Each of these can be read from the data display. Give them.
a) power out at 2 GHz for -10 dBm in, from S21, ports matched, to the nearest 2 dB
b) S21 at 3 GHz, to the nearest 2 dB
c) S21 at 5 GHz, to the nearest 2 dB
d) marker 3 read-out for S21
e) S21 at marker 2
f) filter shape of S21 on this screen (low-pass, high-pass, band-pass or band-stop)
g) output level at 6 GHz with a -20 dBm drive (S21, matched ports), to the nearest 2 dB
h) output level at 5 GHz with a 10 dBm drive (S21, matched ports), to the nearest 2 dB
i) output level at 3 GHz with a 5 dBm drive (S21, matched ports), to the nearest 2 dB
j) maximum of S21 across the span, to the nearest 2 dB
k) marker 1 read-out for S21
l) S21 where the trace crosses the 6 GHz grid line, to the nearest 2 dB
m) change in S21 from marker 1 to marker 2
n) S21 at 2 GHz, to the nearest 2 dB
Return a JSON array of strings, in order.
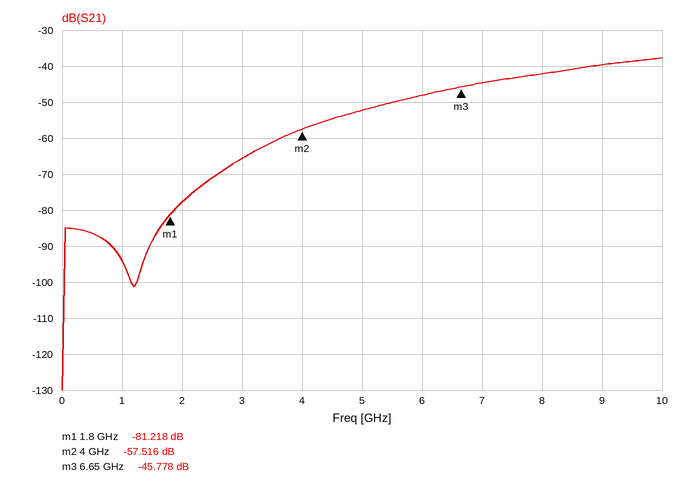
["-88 dBm", "-66 dB", "-52 dB", "-45.778 dB", "-57.516 dB", "high-pass", "-68 dBm", "-42 dBm", "-60 dBm", "-38 dB", "-81.218 dB", "-48 dB", "23.702 dB", "-78 dB"]
